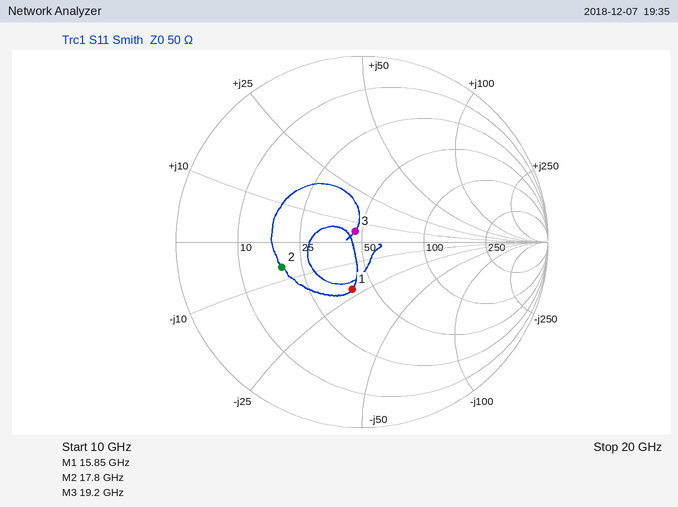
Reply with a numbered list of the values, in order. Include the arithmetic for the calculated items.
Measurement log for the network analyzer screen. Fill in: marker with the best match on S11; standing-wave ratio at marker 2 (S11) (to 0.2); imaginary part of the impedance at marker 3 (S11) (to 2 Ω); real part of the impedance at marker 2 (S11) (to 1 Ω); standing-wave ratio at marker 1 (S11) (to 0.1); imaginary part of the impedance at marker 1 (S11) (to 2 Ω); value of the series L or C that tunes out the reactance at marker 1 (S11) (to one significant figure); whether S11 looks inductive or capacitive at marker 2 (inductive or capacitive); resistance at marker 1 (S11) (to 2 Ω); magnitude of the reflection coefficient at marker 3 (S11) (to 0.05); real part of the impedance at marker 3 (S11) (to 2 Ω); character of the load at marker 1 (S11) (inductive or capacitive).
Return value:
1. marker 3
2. 2.6
3. +6 Ω
4. 19 Ω
5. 1.7
6. -22 Ω
7. L = 22 Ω/(2π × 15.85 GHz) ≈ 221 pH, so 200 pH to one significant figure
8. capacitive
9. 40 Ω
10. 0.05
11. 46 Ω
12. capacitive
